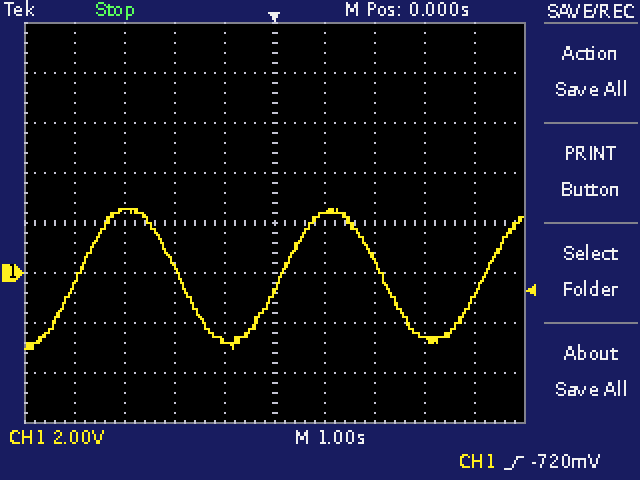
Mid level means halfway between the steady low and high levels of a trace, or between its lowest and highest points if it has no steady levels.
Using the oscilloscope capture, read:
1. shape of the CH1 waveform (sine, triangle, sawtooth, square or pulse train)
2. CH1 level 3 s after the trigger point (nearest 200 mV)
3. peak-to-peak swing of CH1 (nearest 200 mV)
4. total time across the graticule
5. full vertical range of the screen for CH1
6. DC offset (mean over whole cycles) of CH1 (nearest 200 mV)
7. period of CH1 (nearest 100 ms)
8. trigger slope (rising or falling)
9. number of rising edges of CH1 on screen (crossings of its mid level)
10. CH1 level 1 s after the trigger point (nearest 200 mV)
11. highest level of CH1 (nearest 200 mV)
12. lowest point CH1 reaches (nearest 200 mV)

sine
-2.6 V
5.6 V
10 s
16 V
-200 mV
4.1 s
rising
3
2.4 V
2.6 V
-3.0 V
